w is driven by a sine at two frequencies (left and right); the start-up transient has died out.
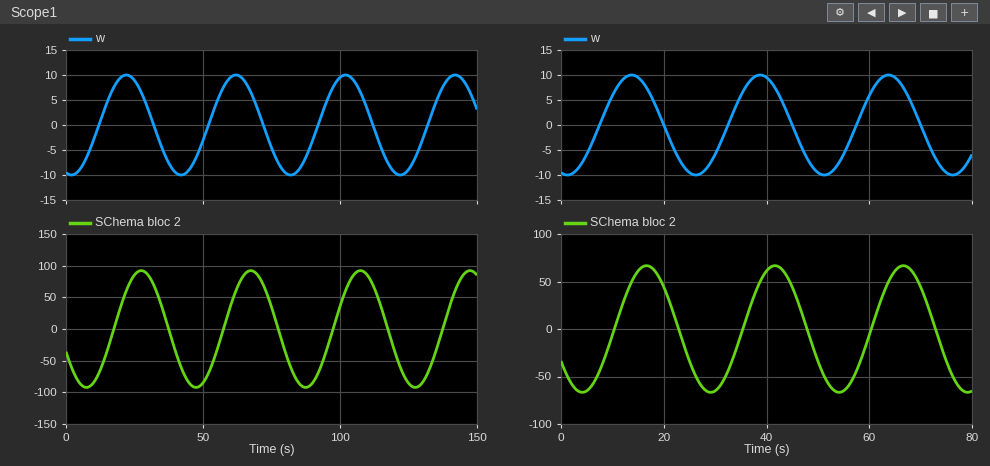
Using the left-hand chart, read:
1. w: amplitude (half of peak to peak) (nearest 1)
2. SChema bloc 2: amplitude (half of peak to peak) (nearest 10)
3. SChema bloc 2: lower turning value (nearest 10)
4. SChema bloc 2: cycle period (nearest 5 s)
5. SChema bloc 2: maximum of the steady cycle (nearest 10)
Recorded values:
10
90
-90
40 s
90
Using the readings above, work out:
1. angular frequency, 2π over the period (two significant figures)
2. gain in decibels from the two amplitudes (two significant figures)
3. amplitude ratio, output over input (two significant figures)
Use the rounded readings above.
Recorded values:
0.16 rad/s
19 dB
9.0
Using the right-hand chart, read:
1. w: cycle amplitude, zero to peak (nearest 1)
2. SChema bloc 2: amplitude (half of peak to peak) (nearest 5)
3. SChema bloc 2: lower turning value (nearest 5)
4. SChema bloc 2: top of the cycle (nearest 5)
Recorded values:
10
65
-65
65
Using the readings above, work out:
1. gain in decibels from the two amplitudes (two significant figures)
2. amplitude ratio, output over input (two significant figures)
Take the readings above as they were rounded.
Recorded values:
16 dB
6.5
